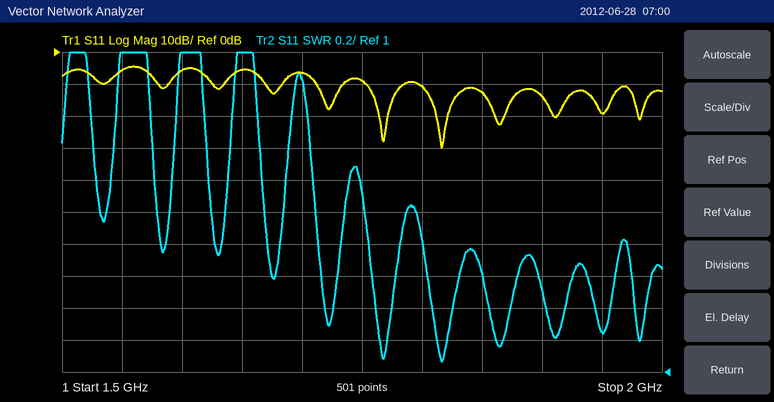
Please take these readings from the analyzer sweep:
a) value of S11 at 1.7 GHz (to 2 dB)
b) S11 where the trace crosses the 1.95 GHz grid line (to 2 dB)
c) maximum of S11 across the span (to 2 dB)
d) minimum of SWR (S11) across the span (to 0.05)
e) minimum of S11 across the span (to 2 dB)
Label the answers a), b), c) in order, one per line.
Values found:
a) -6 dB
b) -20 dB
c) -4 dB
d) 1.05
e) -30 dB
